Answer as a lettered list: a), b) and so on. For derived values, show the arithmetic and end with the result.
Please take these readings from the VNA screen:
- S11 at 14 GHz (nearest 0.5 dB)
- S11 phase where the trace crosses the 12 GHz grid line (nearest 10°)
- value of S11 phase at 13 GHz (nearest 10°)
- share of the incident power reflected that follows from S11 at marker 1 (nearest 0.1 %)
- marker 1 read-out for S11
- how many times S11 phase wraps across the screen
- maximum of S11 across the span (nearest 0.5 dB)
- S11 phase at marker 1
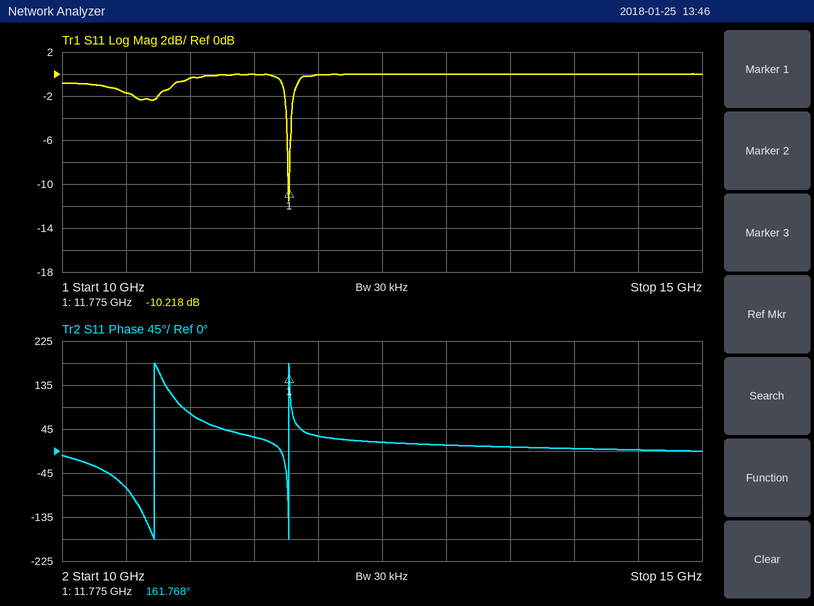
a) 0.0 dB
b) 30°
c) 10°
d) 10^(-10.218/10) ≈ 9.5 %
e) -10.218 dB
f) 2
g) 0.0 dB
h) 161.768°
